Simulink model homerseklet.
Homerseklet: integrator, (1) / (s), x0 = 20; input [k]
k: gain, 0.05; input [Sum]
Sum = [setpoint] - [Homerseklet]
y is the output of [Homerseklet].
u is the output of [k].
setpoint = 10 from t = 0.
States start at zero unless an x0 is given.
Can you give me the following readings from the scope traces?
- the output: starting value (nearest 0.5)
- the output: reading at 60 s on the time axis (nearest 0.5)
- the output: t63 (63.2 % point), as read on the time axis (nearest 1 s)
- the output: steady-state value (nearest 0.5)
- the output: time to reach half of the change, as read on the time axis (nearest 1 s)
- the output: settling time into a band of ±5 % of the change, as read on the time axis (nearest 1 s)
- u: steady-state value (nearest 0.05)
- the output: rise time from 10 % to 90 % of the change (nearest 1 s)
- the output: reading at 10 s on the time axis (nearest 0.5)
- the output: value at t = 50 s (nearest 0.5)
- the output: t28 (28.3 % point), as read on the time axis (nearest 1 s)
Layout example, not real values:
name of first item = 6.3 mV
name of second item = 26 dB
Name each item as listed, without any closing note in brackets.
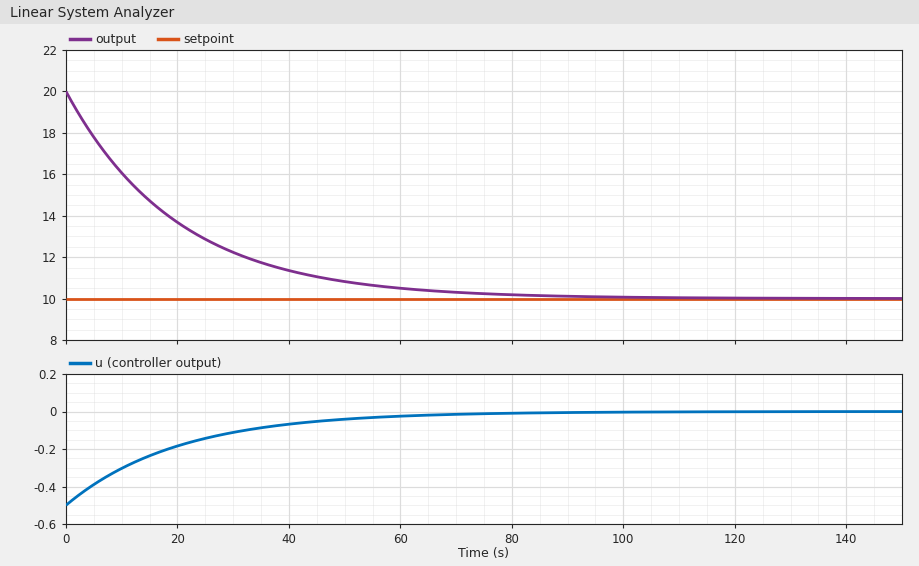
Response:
the output: starting value = 20.0
the output: reading at 60 s on the time axis = 10.5
the output: t63 (63.2 % point), as read on the time axis = 20 s
the output: steady-state value = 10.0
the output: time to reach half of the change, as read on the time axis = 14 s
the output: settling time into a band of ±5 % of the change, as read on the time axis = 60 s
u: steady-state value = 0.00
the output: rise time from 10 % to 90 % of the change = 44 s
the output: reading at 10 s on the time axis = 16.0
the output: value at t = 50 s = 11.0
the output: t28 (28.3 % point), as read on the time axis = 7 s
